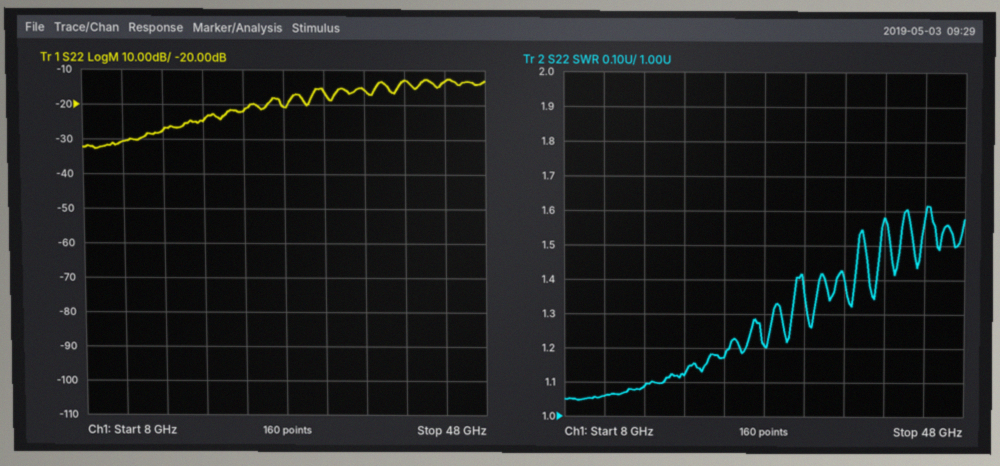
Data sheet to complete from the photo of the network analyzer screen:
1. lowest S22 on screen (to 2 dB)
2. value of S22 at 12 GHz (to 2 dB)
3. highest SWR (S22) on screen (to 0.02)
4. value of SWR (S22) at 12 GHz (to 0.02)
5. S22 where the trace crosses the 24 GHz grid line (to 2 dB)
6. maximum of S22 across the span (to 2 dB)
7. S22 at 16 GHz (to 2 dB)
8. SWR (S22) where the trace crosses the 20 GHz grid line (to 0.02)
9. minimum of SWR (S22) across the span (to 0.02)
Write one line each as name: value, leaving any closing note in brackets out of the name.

lowest S22 on screen: -32 dB
value of S22 at 12 GHz: -30 dB
highest SWR (S22) on screen: 1.62
value of SWR (S22) at 12 GHz: 1.06
S22 where the trace crosses the 24 GHz grid line: -22 dB
maximum of S22 across the span: -12 dB
S22 at 16 GHz: -28 dB
SWR (S22) where the trace crosses the 20 GHz grid line: 1.12
minimum of SWR (S22) across the span: 1.04
